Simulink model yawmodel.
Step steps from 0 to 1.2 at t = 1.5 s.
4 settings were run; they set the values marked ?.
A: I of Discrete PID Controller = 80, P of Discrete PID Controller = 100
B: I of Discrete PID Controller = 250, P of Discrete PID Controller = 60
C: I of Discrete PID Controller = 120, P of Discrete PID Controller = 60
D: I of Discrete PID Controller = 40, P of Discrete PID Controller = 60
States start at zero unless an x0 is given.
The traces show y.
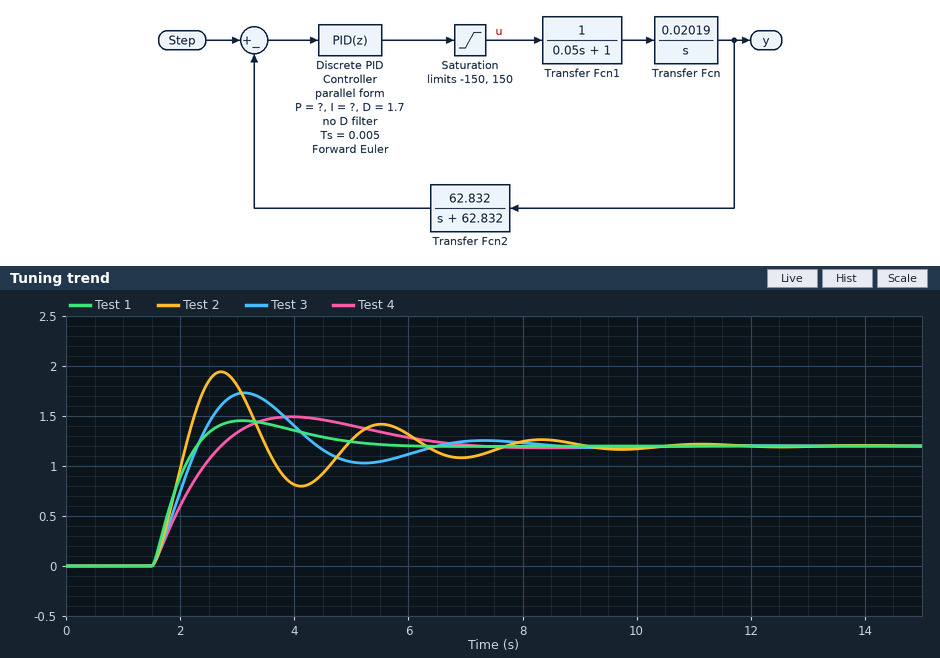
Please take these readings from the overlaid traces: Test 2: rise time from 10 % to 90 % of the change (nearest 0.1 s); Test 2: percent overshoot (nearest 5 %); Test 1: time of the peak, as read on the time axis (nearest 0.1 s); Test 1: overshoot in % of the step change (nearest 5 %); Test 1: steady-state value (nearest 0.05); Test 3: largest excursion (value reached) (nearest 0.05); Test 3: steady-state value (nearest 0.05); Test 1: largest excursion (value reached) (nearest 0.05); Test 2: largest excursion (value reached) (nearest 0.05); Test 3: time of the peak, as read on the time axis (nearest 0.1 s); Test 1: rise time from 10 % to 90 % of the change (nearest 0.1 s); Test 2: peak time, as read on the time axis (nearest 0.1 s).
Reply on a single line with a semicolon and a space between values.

0.4 s; 60 %; 3.1 s; 20 %; 1.20; 1.75; 1.20; 1.45; 1.95; 3.1 s; 0.6 s; 2.7 s
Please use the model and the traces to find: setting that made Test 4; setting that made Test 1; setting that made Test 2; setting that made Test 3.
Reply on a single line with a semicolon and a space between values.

D; A; B; C
